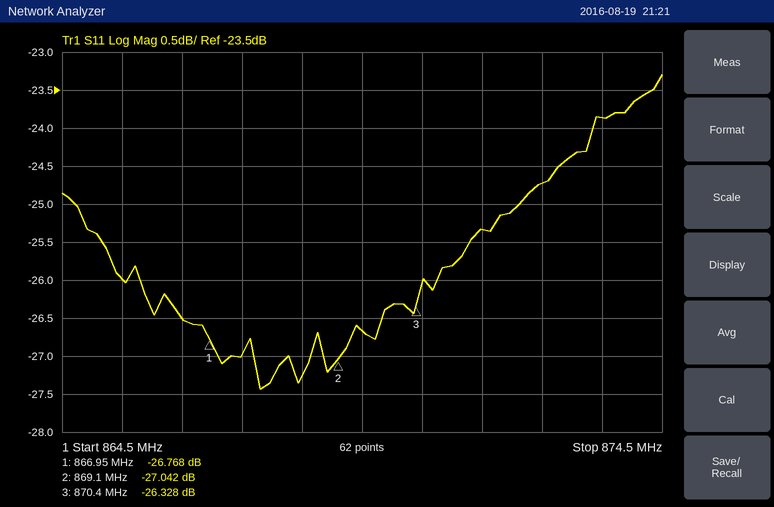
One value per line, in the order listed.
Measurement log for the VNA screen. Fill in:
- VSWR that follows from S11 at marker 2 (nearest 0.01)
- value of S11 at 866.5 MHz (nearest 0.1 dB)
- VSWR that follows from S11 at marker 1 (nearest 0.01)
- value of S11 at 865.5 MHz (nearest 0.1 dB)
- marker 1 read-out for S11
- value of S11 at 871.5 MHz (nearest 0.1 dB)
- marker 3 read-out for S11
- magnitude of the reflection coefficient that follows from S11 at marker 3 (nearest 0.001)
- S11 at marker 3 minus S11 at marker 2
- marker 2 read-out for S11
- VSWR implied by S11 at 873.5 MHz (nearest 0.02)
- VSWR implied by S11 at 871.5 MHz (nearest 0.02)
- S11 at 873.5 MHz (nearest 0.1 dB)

1.09
-26.5 dB
1.10
-26.0 dB
-26.768 dB
-25.3 dB
-26.328 dB
0.048
0.714 dB
-27.042 dB
1.14
1.12
-23.9 dB
